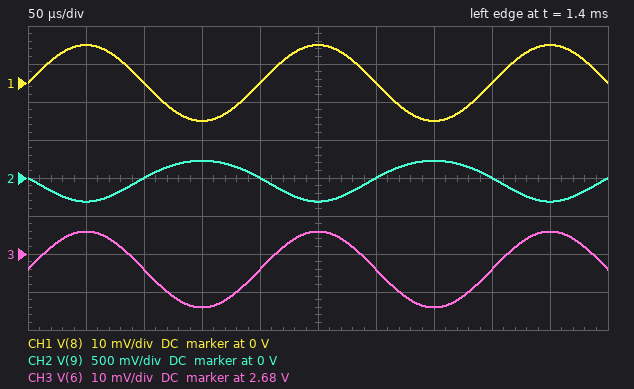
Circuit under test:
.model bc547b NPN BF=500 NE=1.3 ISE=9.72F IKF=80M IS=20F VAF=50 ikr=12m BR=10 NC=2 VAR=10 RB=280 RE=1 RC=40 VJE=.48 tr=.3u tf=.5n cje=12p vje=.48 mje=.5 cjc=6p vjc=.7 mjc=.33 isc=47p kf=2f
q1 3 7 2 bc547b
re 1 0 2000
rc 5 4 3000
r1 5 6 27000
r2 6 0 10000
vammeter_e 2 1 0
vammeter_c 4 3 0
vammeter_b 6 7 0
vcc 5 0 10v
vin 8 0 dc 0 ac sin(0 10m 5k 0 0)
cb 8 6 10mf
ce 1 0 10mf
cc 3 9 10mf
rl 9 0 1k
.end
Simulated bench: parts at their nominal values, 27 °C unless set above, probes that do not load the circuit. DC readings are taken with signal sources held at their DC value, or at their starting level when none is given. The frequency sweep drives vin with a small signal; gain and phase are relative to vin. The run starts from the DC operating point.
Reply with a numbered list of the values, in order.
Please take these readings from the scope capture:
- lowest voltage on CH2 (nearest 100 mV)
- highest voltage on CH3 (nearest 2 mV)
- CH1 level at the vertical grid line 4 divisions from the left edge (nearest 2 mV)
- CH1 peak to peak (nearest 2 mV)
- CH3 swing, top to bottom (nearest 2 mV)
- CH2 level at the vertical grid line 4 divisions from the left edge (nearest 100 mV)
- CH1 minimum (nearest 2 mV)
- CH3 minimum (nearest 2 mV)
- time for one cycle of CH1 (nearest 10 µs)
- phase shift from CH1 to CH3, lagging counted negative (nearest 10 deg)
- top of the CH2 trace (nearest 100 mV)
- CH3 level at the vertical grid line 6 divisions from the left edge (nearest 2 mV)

1. -300 mV
2. 2.686 V
3. 0 V
4. 20 mV
5. 20 mV
6. 0 V
7. -10 mV
8. 2.666 V
9. 200 µs
10. 0 deg
11. 200 mV
12. 2.676 V
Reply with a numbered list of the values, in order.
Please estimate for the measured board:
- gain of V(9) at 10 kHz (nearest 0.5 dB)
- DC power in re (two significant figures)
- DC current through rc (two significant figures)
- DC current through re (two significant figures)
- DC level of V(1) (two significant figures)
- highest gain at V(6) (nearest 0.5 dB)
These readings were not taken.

1. 28.5 dB
2. 2.1 mW
3. 1.0 mA
4. 1.0 mA
5. 2.0 V
6. 0 dB
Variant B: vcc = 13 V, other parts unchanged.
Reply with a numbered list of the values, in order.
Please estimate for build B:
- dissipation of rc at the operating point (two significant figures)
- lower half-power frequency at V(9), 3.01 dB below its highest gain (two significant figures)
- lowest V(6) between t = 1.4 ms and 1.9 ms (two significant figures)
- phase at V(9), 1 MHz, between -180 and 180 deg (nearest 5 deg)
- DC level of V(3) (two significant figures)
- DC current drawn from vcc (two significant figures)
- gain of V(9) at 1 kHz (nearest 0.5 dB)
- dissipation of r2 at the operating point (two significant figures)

1. 6.0 mW
2. 770 mHz
3. 3.5 V
4. 165 deg
5. 8.8 V
6. 1.8 mA
7. 31.0 dB
8. 1.2 mW
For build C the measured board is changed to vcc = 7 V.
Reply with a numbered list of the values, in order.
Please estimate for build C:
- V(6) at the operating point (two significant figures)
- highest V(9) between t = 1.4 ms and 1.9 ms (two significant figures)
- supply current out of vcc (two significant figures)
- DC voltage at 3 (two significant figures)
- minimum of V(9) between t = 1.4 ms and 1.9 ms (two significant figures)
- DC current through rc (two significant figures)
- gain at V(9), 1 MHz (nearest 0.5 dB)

1. 1.9 V
2. 140 mV
3. 810 µA
4. 5.1 V
5. -200 mV
6. 620 µA
7. 24.5 dB
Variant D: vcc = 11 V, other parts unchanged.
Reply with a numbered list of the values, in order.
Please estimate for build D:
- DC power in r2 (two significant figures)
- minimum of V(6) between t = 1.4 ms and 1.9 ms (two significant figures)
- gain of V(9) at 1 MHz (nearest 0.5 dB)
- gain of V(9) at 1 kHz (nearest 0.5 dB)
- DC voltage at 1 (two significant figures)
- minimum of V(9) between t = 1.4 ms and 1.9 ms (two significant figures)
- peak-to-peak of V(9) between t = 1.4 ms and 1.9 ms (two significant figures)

1. 870 µW
2. 2.9 V
3. 29.0 dB
4. 29.5 dB
5. 2.3 V
6. -350 mV
7. 600 mV
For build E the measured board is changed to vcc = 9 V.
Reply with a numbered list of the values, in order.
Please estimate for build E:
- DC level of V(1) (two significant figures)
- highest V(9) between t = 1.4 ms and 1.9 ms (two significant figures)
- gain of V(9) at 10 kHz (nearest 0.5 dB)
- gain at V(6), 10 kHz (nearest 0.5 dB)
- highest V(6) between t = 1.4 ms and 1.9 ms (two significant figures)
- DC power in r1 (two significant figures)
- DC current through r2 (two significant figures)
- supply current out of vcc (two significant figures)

1. 1.8 V
2. 200 mV
3. 27.5 dB
4. 0 dB
5. 2.4 V
6. 1.6 mW
7. 240 µA
8. 1.1 mA
